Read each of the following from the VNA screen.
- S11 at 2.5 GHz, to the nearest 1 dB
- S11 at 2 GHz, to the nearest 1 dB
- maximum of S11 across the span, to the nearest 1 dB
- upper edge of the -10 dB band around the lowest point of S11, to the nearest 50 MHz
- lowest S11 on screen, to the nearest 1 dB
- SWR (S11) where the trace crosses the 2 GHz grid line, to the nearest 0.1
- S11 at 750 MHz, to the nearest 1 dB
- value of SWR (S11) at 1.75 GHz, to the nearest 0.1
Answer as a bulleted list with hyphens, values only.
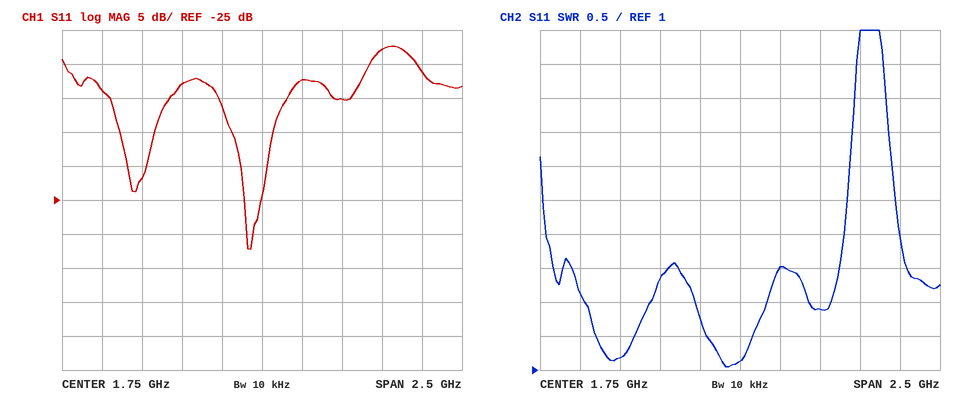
- -3 dB
- -7 dB
- -2 dB
- 1.90 GHz
- -32 dB
- 2.5
- -9 dB
- 1.1
